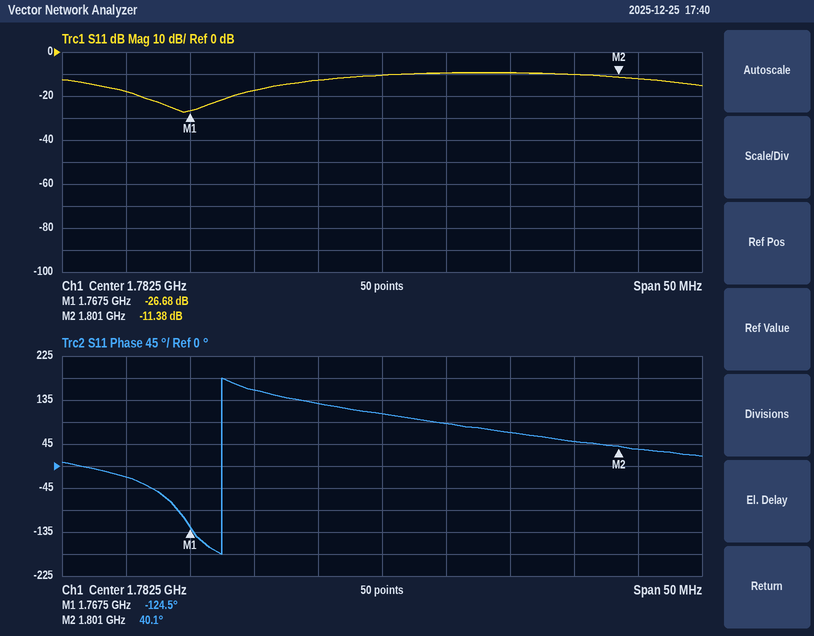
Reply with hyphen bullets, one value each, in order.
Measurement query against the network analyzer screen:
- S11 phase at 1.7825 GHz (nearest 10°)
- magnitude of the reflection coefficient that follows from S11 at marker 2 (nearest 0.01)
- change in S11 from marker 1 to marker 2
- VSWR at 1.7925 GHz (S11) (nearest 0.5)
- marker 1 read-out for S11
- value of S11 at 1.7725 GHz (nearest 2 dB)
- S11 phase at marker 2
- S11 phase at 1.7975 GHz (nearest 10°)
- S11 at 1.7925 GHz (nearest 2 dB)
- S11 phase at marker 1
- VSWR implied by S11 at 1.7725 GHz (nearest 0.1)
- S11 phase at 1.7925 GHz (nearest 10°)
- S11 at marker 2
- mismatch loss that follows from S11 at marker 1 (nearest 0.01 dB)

- 110°
- 0.27
- 15.30 dB
- 2.0
- -26.68 dB
- -18 dB
- 40.1°
- 50°
- -10 dB
- -124.5°
- 1.3
- 70°
- -11.38 dB
- 0.01 dB
